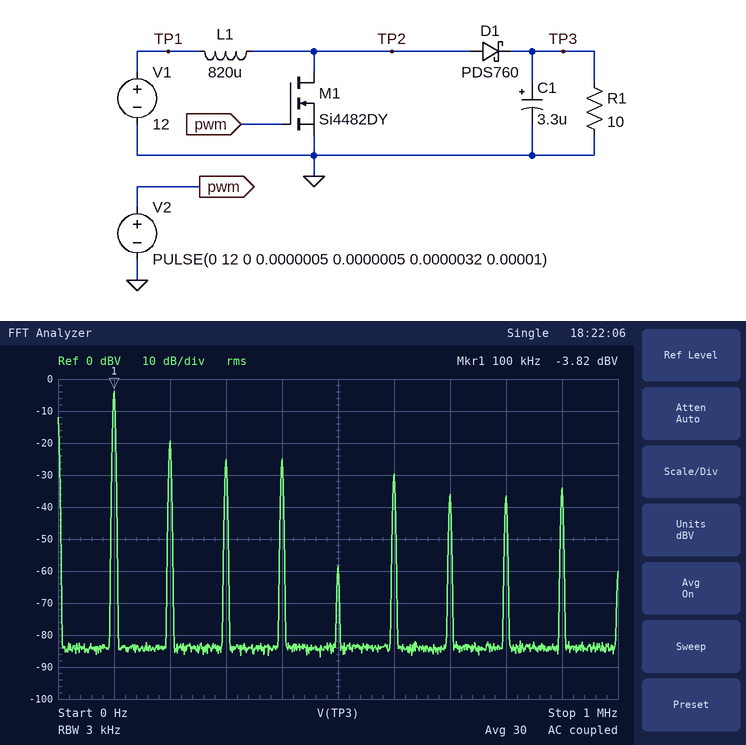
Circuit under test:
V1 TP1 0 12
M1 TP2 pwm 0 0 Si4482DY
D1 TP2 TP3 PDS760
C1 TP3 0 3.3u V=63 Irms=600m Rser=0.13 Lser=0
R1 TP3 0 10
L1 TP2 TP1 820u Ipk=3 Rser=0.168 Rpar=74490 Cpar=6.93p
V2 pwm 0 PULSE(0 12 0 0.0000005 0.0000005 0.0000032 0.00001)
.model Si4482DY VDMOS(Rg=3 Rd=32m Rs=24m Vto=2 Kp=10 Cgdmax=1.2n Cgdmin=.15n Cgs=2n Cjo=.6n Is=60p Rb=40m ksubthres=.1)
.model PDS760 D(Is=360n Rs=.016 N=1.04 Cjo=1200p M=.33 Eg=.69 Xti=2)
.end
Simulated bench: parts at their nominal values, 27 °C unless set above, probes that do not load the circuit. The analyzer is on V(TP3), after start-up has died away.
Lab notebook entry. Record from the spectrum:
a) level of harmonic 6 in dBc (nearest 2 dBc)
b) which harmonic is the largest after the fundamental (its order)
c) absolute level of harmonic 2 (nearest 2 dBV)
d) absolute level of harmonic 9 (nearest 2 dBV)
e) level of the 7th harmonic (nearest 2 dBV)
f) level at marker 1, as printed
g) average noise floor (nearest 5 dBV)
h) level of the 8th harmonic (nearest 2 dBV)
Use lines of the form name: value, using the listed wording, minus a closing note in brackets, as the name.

level of harmonic 6 in dBc: -26 dBc
which harmonic is the largest after the fundamental: 2
absolute level of harmonic 2: -20 dBV
absolute level of harmonic 9: -34 dBV
level of the 7th harmonic: -36 dBV
level at marker 1, as printed: -3.82 dBV
average noise floor: -85 dBV
level of the 8th harmonic: -36 dBV
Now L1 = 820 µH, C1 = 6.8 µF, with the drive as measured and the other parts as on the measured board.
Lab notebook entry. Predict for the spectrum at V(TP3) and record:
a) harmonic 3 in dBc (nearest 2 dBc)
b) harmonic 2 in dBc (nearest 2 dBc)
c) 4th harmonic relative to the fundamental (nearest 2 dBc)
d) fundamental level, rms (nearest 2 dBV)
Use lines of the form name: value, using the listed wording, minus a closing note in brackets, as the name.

harmonic 3 in dBc: -18 dBc
harmonic 2 in dBc: -14 dBc
4th harmonic relative to the fundamental: -18 dBc
fundamental level, rms: -10 dBV
